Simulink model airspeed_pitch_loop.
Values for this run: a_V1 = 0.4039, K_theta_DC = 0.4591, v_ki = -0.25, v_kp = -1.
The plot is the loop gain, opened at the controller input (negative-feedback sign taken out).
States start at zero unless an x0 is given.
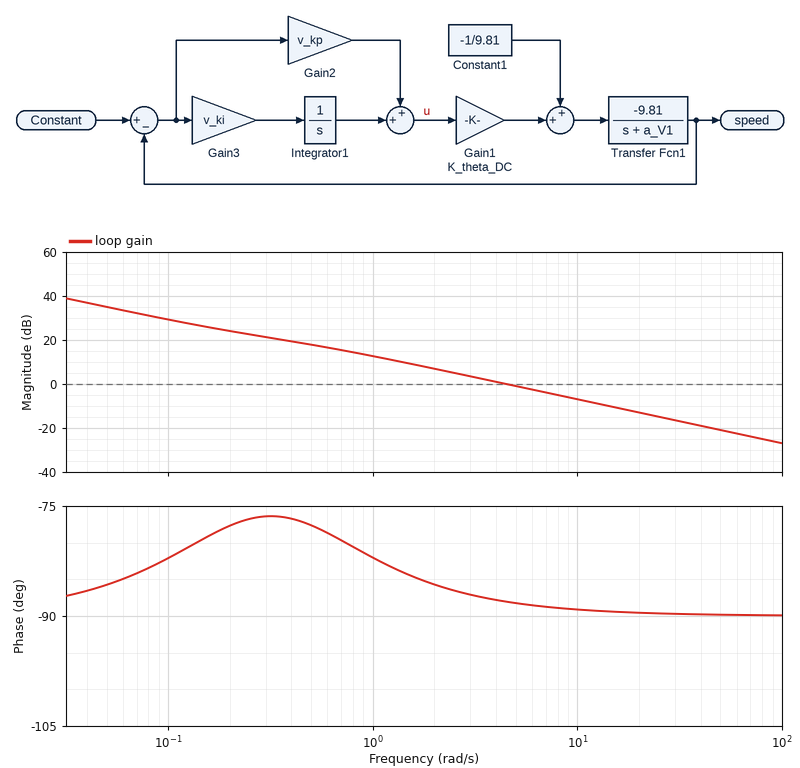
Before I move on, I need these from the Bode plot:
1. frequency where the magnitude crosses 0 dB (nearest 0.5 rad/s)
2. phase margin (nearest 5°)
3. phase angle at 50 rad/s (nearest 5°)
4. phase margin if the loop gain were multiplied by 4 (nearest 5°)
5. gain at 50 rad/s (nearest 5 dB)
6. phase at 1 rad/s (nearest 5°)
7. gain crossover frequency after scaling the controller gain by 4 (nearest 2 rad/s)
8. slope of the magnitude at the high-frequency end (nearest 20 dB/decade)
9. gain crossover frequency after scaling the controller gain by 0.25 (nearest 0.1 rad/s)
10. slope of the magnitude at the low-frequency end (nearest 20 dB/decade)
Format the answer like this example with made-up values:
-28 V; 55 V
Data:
4.5 rad/s; 90°; -90°; 90°; -20 dB; -80°; 18 rad/s; -20 dB/decade; 1.1 rad/s; -20 dB/decade
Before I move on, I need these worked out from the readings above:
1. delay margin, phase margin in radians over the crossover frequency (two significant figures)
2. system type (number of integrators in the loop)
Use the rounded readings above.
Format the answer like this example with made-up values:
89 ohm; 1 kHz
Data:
0.35 s; 1
